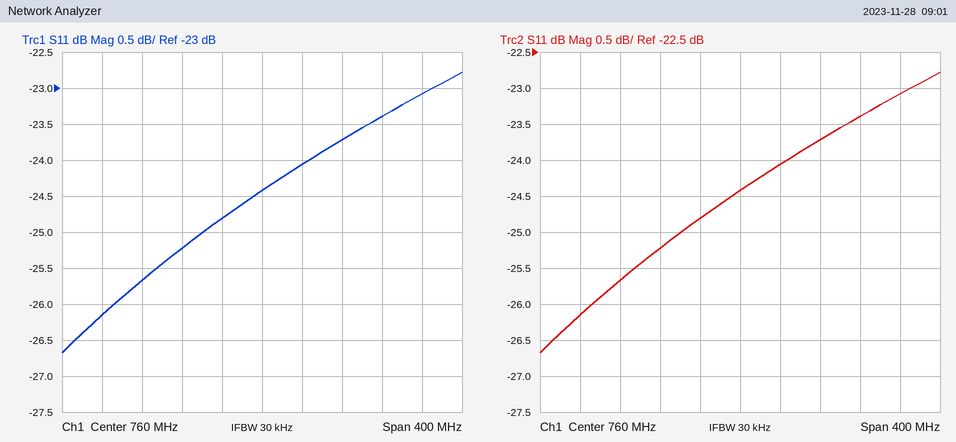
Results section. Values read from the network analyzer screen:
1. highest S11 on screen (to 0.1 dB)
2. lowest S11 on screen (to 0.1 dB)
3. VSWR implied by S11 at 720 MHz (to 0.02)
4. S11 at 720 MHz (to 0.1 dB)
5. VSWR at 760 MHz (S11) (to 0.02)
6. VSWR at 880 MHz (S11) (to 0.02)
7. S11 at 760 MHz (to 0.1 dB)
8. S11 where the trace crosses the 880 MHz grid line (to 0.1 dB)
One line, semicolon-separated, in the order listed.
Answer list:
-22.8 dB; -26.7 dB; 1.12; -24.8 dB; 1.12; 1.14; -24.4 dB; -23.4 dB
